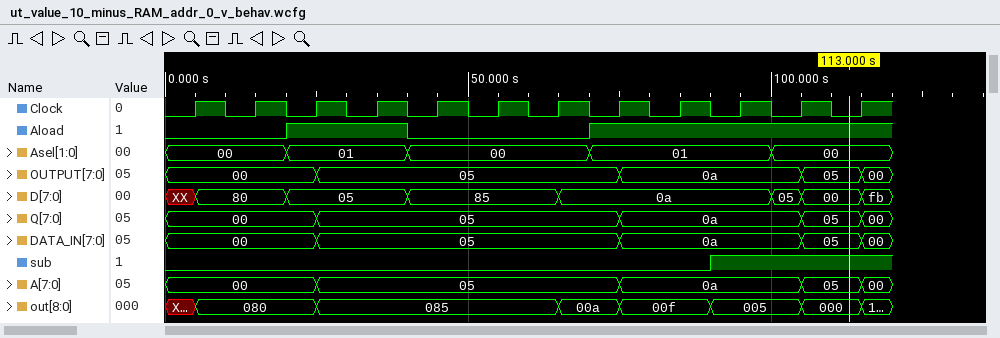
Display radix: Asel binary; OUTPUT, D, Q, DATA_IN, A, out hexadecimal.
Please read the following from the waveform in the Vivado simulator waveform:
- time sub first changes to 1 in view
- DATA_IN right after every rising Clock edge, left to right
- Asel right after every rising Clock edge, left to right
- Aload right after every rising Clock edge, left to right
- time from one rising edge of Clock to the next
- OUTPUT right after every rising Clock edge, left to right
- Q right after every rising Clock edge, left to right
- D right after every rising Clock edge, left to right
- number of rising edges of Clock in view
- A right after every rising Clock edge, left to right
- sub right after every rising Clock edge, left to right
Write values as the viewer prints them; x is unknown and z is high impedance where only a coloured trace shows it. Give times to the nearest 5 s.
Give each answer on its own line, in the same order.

90 s
00, 00, 05, 05, 05, 05, 05, 0a, 0a, 0a, 05, 00
00, 00, 01, 01, 00, 00, 00, 01, 01, 01, 00, 00
0 0 1 1 0 0 0 1 1 1 1 1
10 s
00, 00, 05, 05, 05, 05, 05, 0a, 0a, 0a, 05, 00
00, 00, 05, 05, 05, 05, 05, 0a, 0a, 0a, 05, 00
80, 80, 05, 05, 85, 85, 0a, 0a, 0a, 0a, 00, fb
12
00, 00, 05, 05, 05, 05, 05, 0a, 0a, 0a, 05, 00
0 0 0 0 0 0 0 0 0 1 1 1
